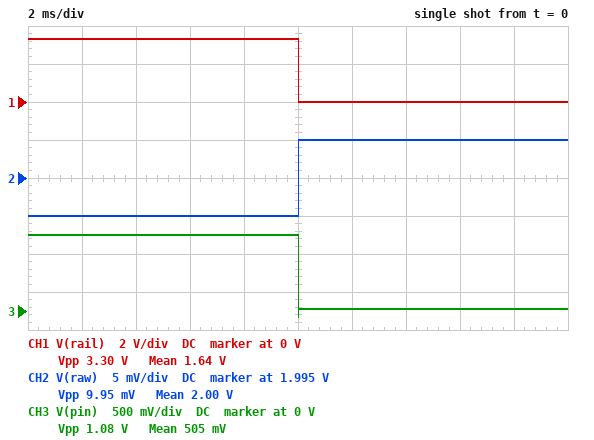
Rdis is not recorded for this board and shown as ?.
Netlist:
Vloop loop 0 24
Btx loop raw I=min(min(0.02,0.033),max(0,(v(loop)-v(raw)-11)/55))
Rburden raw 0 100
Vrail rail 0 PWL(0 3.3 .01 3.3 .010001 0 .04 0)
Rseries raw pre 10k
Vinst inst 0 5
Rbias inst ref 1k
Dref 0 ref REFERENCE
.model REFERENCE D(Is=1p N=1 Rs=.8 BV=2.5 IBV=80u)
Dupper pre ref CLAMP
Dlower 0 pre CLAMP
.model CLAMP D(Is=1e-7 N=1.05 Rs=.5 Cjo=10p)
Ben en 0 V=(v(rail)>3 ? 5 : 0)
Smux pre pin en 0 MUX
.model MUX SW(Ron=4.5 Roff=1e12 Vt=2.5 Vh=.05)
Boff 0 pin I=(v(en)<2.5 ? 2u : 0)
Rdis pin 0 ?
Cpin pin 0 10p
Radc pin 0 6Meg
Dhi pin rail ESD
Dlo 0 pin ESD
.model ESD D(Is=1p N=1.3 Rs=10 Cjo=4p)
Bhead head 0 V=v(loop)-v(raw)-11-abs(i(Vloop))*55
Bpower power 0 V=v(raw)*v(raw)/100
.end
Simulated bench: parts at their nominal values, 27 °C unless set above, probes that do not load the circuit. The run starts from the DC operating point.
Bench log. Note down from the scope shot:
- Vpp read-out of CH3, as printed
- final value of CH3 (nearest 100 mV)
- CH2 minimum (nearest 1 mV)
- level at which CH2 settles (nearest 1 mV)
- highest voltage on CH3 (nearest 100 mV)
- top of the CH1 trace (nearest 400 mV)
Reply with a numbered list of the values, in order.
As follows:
1. 1.08 V
2. 0 V
3. 1.990 V
4. 2.000 V
5. 1.0 V
6. 3.2 V
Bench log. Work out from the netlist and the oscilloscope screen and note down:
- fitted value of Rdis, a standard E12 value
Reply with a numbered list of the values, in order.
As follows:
1. 10 kΩ
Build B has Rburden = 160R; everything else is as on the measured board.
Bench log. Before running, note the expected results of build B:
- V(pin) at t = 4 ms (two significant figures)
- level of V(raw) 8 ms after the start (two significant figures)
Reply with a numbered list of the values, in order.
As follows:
1. 1.6 V
2. 3.2 V
